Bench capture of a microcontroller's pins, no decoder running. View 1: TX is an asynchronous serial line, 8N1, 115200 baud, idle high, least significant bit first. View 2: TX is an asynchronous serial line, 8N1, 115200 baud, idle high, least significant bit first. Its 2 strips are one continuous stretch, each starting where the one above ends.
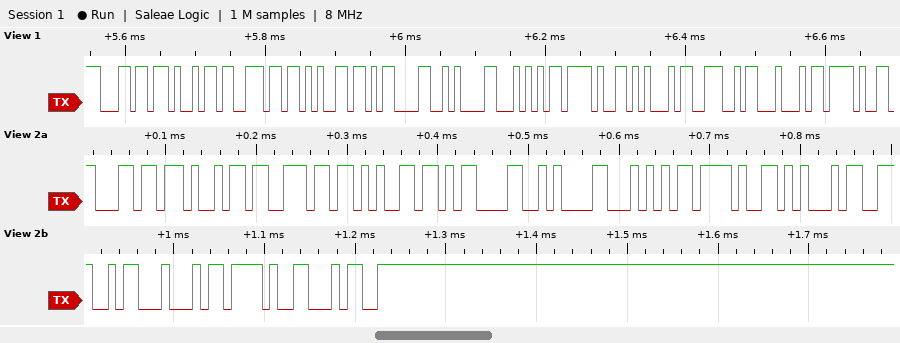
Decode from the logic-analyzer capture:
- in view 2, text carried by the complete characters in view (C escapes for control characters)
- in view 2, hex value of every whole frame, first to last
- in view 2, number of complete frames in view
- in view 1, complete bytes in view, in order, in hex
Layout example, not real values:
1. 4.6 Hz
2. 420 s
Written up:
1. "line\r\nT/END/4"
2. 6C 69 6E 65 0D 0A 54 2F 45 4E 44 2F 34
3. 13
4. 0x6C 0x69 0x6E 0x65 0x0D 0x0A 0x54 0x2F 0x45 0x4E 0x44 0x2F
